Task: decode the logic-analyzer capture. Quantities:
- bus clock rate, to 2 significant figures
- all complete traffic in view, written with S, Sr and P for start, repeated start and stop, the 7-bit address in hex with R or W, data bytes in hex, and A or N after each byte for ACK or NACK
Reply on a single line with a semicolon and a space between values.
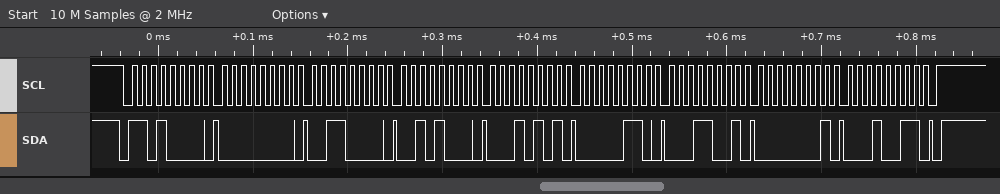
100 kHz; S 68W A 00 A 30 A 28 A 15 A 06 A 19 A 01 A 13 A P
